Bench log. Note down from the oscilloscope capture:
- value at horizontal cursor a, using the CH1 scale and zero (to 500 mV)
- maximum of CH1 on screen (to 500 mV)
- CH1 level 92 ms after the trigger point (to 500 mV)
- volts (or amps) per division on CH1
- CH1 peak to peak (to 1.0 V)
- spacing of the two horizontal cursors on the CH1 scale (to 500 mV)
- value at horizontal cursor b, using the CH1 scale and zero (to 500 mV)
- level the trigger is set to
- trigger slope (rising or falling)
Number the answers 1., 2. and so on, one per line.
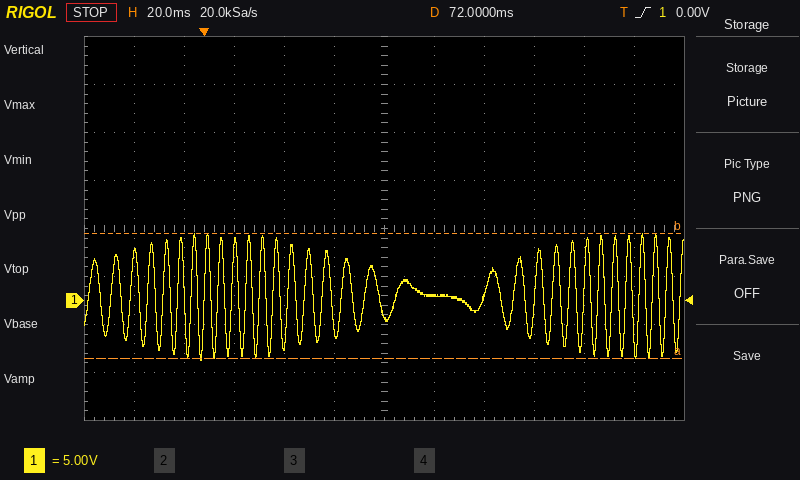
1. -6.0 V
2. 7.0 V
3. 500 mV
4. 5 V
5. 13.0 V
6. 13.0 V
7. 7.0 V
8. 0.00 V
9. rising
